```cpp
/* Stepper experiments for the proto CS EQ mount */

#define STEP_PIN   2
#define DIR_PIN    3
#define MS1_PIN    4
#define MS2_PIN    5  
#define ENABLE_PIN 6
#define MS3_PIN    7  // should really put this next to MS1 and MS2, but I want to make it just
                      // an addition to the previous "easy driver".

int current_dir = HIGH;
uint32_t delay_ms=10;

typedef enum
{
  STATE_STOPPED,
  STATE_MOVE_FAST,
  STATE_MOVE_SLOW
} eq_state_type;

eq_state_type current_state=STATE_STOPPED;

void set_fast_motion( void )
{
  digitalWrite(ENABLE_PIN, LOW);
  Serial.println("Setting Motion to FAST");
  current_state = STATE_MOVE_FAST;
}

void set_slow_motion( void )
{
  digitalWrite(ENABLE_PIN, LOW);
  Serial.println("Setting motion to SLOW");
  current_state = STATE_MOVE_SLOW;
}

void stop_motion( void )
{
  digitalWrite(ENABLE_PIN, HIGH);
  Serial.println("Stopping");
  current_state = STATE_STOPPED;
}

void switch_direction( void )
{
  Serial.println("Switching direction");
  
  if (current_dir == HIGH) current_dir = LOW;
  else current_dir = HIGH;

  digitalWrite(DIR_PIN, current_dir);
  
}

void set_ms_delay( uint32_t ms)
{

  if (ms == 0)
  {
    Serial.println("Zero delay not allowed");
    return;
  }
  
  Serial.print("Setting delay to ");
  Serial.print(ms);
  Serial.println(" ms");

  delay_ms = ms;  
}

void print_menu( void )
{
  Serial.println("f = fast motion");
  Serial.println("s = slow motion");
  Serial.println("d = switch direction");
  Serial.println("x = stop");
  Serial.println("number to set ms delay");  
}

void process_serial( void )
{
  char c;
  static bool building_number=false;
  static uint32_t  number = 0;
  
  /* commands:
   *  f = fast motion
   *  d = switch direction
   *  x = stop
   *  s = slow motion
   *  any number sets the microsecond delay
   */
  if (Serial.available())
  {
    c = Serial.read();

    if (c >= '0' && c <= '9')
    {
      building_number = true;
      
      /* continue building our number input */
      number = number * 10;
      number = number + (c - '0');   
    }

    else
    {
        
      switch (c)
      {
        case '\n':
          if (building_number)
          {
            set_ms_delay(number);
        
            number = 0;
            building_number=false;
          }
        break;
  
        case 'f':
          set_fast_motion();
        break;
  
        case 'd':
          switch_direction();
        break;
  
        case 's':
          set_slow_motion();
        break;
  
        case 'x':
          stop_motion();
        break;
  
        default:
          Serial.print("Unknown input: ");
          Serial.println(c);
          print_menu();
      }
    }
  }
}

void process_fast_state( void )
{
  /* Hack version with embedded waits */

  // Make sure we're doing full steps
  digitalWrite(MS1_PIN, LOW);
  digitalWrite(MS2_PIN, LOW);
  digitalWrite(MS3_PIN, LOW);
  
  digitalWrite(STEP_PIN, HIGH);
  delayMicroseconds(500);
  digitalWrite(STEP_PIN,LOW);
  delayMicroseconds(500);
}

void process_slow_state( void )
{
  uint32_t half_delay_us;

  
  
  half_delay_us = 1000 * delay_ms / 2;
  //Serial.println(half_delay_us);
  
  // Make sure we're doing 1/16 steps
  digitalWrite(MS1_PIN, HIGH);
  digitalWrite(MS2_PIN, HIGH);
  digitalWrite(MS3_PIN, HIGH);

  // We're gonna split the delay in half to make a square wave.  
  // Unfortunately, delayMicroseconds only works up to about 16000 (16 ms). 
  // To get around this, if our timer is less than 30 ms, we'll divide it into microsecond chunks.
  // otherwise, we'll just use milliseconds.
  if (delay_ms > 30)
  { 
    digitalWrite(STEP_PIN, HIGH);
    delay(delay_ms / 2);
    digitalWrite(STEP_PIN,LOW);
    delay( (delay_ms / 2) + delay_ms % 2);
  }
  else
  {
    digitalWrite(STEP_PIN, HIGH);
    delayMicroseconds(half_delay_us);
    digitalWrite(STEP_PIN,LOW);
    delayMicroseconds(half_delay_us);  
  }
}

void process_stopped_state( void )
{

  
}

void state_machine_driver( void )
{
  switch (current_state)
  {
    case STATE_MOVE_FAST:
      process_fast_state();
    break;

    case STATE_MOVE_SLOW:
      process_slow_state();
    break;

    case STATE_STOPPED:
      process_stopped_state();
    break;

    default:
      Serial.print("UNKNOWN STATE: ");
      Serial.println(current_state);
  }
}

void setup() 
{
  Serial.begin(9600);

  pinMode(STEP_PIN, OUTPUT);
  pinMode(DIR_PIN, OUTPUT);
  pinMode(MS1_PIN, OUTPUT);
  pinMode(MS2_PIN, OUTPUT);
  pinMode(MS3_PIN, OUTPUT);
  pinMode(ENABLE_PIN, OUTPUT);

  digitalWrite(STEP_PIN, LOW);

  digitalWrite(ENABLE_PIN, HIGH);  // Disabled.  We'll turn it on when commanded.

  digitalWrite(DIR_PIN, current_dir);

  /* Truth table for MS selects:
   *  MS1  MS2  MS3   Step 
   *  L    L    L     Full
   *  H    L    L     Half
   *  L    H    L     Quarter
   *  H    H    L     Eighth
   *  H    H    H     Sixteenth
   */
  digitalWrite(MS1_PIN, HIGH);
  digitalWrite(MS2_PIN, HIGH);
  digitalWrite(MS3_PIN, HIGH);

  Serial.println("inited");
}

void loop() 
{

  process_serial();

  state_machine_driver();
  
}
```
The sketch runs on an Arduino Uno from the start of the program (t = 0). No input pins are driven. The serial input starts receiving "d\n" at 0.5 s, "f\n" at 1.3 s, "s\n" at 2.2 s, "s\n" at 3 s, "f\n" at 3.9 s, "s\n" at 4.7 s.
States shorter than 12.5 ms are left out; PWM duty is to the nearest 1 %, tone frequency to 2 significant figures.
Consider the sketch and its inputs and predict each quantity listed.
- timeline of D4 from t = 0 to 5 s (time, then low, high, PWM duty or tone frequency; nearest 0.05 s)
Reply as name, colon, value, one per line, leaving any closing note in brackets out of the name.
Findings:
timeline of D4 from t = 0 to 5 s: 0 s high; 1.3 s low; 2.2 s high; 3.9 s low; 4.7 s high
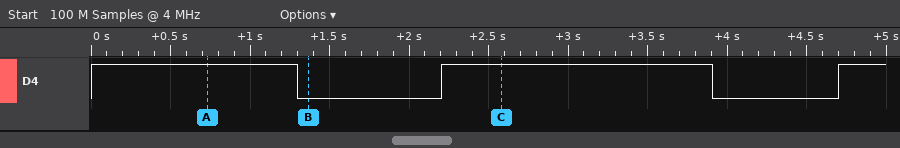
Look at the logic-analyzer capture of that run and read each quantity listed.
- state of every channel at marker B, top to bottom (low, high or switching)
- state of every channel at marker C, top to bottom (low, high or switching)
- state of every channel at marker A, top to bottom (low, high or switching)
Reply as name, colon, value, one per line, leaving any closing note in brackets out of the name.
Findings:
state of every channel at marker B, top to bottom: D4 low
state of every channel at marker C, top to bottom: D4 high
state of every channel at marker A, top to bottom: D4 high
